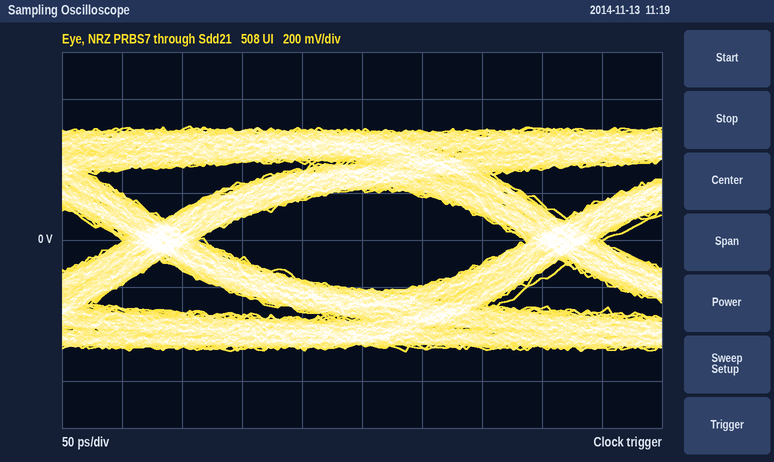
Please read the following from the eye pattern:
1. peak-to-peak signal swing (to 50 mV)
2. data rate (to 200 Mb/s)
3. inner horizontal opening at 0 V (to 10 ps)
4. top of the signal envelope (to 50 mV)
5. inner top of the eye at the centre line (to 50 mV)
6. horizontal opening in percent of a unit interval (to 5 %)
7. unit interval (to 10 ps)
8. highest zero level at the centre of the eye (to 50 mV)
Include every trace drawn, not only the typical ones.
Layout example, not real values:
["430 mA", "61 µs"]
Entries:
["950 mV", "3.0 Gb/s", "270 ps", "500 mV", "200 mV", "80 %", "330 ps", "-200 mV"]
